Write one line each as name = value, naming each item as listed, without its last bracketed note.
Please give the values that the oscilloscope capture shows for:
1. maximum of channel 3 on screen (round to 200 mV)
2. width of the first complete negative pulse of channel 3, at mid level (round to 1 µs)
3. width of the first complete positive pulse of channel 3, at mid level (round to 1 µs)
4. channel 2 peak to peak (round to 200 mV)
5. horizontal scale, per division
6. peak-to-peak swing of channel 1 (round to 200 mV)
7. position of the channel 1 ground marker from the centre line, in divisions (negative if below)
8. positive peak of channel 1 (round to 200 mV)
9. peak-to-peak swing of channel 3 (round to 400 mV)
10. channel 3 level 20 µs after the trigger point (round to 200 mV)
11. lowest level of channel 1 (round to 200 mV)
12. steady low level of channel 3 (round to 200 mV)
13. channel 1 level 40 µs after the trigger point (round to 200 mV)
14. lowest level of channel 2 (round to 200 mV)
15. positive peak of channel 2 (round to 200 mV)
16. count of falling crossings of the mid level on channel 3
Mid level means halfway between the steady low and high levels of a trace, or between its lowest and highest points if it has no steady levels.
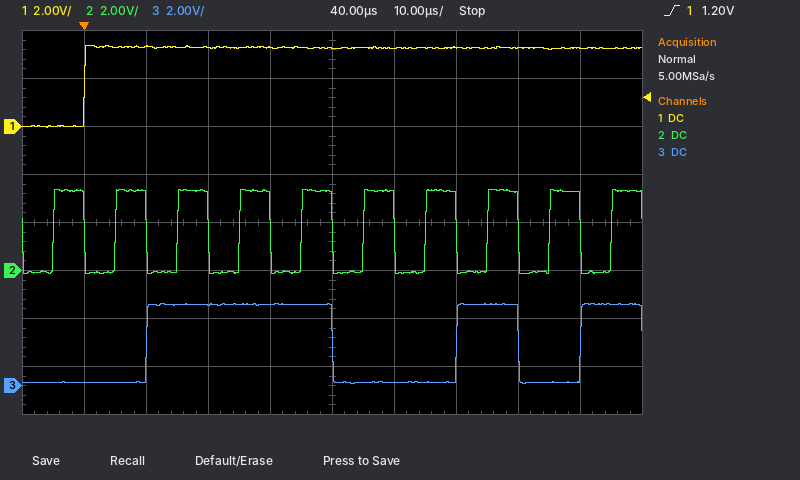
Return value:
maximum of channel 3 on screen = 3.4 V
width of the first complete negative pulse of channel 3, at mid level = 20 µs
width of the first complete positive pulse of channel 3, at mid level = 30 µs
channel 2 peak to peak = 3.6 V
horizontal scale, per division = 10 µs
peak-to-peak swing of channel 1 = 3.4 V
position of the channel 1 ground marker from the centre line, in divisions = +2.0 div
positive peak of channel 1 = 3.4 V
peak-to-peak swing of channel 3 = 3.2 V
channel 3 level 20 µs after the trigger point = 3.4 V
lowest level of channel 1 = 0.0 V
steady low level of channel 3 = 200 mV
channel 1 level 40 µs after the trigger point = 3.2 V
lowest level of channel 2 = -200 mV
positive peak of channel 2 = 3.4 V
count of falling crossings of the mid level on channel 3 = 2
